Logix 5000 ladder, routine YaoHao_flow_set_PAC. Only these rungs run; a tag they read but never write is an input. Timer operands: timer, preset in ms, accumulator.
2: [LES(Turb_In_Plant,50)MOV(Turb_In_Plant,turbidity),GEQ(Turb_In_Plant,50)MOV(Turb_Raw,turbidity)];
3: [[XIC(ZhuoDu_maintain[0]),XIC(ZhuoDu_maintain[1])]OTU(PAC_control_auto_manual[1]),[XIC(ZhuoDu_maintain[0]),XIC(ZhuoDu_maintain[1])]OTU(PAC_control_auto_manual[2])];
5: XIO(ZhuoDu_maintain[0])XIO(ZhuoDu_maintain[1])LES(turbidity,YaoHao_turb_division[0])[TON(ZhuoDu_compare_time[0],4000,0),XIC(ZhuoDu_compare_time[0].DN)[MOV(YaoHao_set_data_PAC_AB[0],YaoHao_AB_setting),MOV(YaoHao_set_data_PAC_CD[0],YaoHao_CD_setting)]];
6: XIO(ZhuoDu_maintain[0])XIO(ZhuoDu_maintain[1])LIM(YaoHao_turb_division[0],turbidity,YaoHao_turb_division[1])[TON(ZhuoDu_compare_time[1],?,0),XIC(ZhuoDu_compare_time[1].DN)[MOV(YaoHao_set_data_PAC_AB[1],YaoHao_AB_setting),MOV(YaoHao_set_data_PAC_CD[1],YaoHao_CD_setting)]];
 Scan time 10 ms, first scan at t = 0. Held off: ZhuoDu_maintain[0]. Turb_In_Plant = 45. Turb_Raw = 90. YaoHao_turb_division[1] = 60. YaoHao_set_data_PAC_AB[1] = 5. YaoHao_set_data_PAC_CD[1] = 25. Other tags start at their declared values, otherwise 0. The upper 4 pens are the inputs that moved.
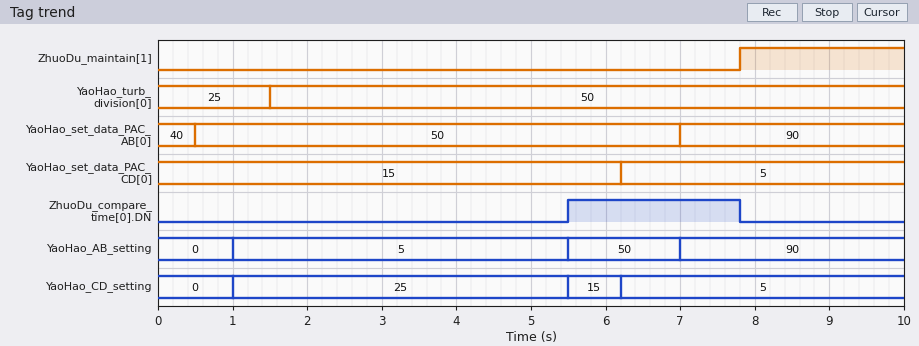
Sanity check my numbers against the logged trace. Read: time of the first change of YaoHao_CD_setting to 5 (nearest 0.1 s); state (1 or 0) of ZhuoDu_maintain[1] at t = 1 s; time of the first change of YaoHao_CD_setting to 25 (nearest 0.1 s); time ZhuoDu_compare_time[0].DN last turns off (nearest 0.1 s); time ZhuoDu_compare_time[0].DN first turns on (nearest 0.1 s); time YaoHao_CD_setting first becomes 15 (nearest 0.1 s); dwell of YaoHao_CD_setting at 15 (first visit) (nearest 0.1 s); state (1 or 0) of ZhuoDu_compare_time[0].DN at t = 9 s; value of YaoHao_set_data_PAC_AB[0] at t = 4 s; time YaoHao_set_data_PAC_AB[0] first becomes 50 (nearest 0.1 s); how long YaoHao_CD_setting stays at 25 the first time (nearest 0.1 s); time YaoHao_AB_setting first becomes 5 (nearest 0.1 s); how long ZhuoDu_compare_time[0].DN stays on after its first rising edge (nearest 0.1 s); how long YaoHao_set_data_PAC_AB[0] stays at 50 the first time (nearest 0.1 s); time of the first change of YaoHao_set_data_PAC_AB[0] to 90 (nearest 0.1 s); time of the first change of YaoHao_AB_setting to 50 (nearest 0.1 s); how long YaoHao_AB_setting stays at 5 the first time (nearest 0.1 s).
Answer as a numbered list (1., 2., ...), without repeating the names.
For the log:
1. 6.2 s
2. 0
3. 1.0 s
4. 7.8 s
5. 5.5 s
6. 5.5 s
7. 0.7 s
8. 0
9. 50
10. 0.5 s
11. 4.5 s
12. 1.0 s
13. 2.3 s
14. 6.5 s
15. 7.0 s
16. 5.5 s
17. 4.5 s
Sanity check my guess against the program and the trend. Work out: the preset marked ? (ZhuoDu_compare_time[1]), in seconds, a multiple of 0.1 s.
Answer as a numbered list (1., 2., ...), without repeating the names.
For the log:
1. 1.0 s
